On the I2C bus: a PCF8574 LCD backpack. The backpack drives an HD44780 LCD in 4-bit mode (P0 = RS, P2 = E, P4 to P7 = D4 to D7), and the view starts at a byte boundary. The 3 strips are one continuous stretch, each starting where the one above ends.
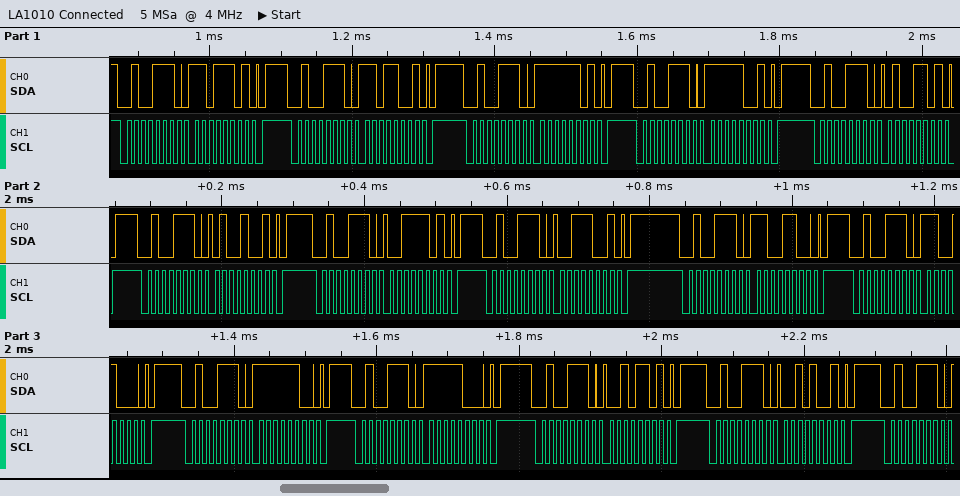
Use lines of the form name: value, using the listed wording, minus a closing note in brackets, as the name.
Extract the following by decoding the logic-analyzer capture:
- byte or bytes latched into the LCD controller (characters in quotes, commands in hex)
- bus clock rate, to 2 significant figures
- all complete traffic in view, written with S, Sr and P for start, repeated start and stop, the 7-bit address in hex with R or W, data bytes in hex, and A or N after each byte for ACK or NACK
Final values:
byte or bytes latched into the LCD controller: data 0xDF 'C' 0xCF
bus clock rate, to 2 significant figures: 100 kHz
all complete traffic in view, written with S, Sr and P for start, repeated start and stop, the 7-bit address in hex with R or W, data bytes in hex, and A or N after each byte for ACK or NACK: S 27W A DD A P S 27W A D9 A P S 27W A FD A P S 27W A F9 A P S 27W A 4D A P S 27W A 49 A P S 27W A 3D A P S 27W A 39 A P S 27W A CC A P S 27W A C8 A P S 27W A FC A P S 27W A F8 A P S 27W A 2D A P S 27W A 29 A P S 27W A
